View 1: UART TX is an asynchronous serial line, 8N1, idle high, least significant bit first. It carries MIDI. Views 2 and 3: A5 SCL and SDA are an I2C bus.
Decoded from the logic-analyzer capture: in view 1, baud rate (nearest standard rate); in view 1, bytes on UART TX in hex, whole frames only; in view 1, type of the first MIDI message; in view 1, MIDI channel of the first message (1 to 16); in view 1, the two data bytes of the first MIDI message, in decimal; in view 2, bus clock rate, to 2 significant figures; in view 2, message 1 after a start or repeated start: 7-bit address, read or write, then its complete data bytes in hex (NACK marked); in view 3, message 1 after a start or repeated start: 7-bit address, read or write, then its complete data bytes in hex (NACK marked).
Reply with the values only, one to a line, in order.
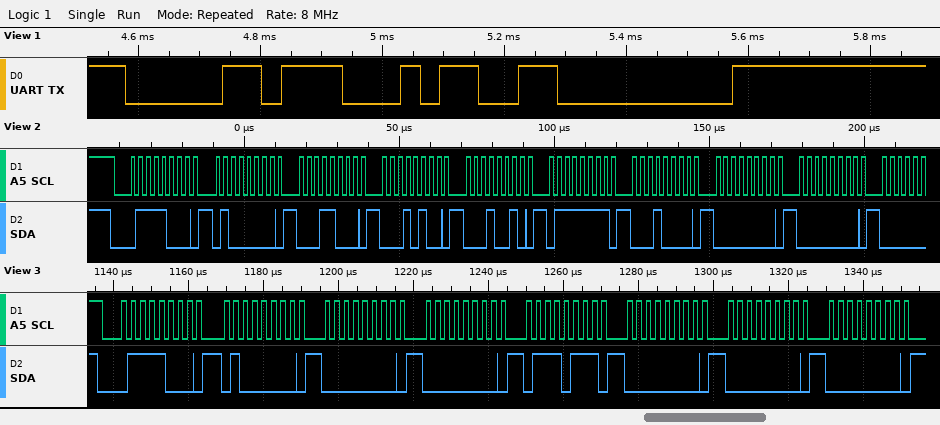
31250 baud
0xB0 0x34 0x00
Control Change
1
52, 0
400 kHz
0x3C write: 40 18 14 12 7F 10 00 00
0x3C write: 40 00 00 77 00 00 00
